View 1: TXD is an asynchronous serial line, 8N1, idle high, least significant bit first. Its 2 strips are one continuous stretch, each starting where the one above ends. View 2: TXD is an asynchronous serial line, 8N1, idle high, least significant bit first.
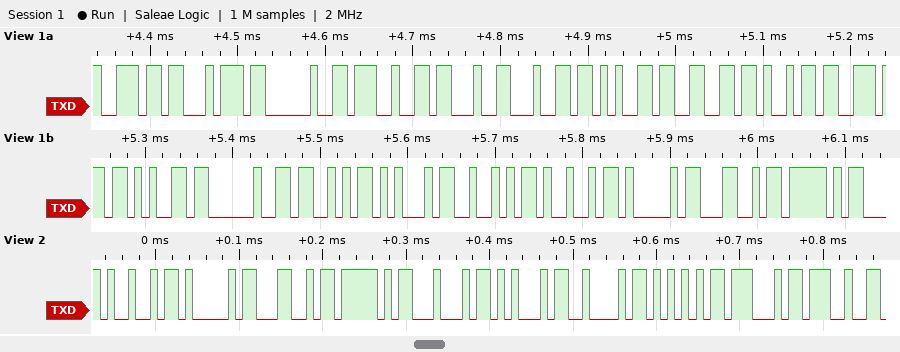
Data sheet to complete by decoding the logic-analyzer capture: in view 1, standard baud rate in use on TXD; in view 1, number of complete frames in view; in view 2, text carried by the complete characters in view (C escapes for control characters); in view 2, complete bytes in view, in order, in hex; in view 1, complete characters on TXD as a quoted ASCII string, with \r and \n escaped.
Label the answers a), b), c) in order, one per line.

a) 115200 baud
b) 19
c) "IAL_DEBUG'"
d) 0x49 0x41 0x4C 0x5F 0x44 0x45 0x42 0x55 0x47 0x27
e) "nt '#define SERIAL_"
